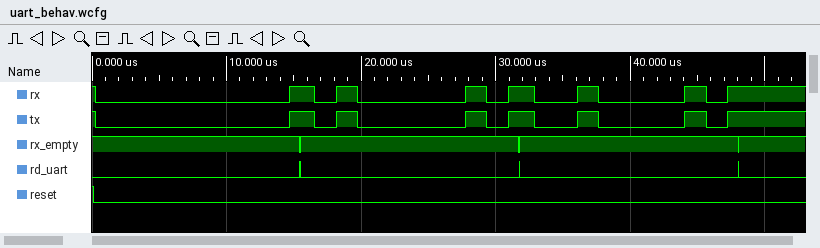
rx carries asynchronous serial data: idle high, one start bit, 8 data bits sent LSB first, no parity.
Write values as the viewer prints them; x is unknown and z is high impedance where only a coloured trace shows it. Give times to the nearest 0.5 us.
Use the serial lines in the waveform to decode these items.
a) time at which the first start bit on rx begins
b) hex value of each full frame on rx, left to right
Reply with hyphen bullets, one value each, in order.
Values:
- 0 us
- 00, 41, 42
